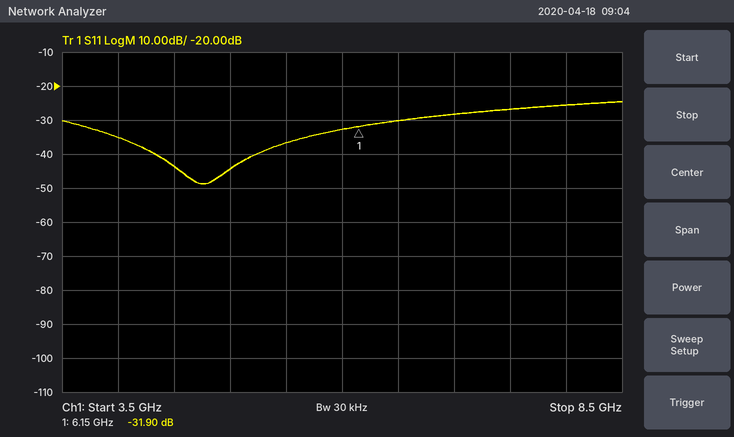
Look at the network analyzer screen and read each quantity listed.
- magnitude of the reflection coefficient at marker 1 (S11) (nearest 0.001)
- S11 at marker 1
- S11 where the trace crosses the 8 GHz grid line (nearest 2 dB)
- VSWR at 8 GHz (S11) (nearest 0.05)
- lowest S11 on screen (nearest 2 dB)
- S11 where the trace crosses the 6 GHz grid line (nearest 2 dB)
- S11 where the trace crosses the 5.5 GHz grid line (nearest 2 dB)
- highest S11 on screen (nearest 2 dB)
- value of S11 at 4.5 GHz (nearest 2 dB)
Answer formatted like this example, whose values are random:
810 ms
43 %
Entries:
0.025
-31.90 dB
-26 dB
1.10
-48 dB
-32 dB
-36 dB
-24 dB
-44 dB
